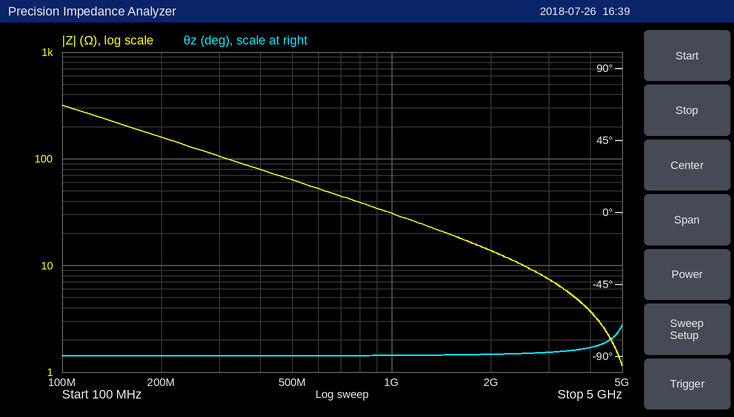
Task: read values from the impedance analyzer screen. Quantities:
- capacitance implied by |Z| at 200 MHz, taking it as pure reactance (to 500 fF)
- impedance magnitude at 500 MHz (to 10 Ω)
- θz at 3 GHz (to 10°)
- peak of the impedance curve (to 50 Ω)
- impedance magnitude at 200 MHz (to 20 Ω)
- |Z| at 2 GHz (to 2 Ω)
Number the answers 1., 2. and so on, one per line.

1. 5.0 pF
2. 60 Ω
3. -90°
4. 300 Ω
5. 160 Ω
6. 14 Ω
